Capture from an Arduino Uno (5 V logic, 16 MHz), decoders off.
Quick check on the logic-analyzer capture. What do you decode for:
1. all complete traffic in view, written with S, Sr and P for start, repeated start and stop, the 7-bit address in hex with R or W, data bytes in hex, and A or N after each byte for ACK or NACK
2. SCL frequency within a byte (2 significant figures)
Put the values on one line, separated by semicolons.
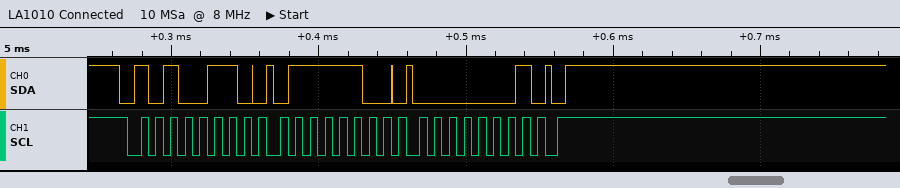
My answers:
S 53W A 7C A 01 A P; 100 kHz
